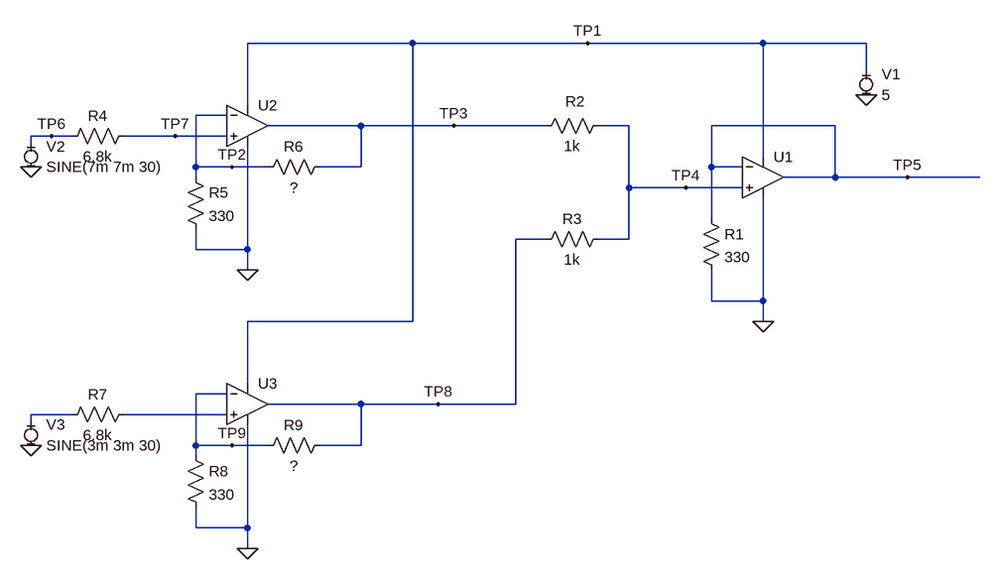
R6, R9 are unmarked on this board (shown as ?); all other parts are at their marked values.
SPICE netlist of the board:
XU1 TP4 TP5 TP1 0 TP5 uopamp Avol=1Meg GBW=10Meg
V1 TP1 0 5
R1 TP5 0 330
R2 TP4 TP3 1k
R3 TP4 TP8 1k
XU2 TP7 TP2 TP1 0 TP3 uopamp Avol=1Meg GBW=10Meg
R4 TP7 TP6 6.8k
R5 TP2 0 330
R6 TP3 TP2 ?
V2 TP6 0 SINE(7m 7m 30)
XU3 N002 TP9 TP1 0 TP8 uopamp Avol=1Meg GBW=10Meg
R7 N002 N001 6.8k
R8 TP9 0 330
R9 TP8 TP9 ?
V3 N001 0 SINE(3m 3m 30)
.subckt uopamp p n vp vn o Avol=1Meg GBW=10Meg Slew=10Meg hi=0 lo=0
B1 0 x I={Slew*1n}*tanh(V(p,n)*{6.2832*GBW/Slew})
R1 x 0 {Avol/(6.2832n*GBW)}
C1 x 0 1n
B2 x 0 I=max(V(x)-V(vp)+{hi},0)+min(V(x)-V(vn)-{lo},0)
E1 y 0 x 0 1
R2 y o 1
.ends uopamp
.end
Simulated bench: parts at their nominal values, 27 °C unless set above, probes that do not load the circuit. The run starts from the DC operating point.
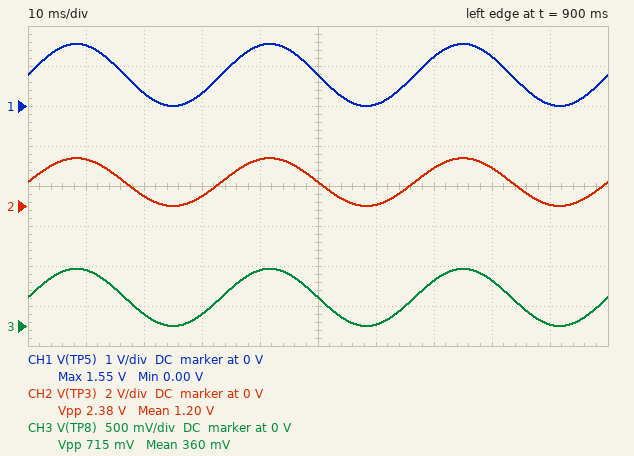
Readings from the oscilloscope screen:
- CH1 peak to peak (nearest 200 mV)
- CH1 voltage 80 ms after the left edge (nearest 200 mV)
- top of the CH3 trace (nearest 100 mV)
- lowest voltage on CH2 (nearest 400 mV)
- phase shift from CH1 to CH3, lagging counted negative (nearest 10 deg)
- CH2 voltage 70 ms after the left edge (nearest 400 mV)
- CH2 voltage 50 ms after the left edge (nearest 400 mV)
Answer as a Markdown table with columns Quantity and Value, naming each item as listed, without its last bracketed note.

| Quantity | Value |
|---|---|
| CH1 peak to peak | 1.6 V |
| CH1 voltage 80 ms after the left edge | 1.2 V |
| top of the CH3 trace | 700 mV |
| lowest voltage on CH2 | 0 V |
| phase shift from CH1 to CH3, lagging counted negative | 0 deg |
| CH2 voltage 70 ms after the left edge | 2.0 V |
| CH2 voltage 50 ms after the left edge | 1.2 V |
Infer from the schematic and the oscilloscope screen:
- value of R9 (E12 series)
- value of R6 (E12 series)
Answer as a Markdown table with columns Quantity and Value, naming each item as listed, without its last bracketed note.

| Quantity | Value |
|---|---|
| value of R9 | 39 kΩ |
| value of R6 | 56 kΩ |
